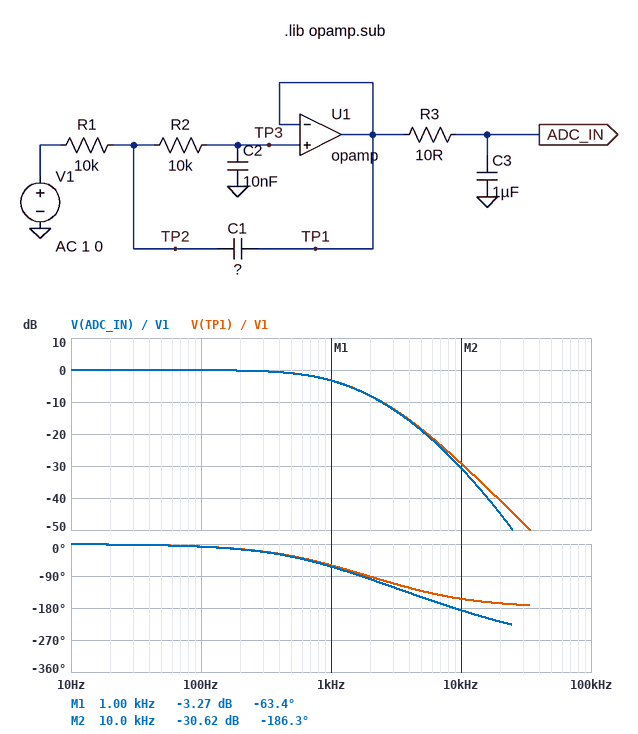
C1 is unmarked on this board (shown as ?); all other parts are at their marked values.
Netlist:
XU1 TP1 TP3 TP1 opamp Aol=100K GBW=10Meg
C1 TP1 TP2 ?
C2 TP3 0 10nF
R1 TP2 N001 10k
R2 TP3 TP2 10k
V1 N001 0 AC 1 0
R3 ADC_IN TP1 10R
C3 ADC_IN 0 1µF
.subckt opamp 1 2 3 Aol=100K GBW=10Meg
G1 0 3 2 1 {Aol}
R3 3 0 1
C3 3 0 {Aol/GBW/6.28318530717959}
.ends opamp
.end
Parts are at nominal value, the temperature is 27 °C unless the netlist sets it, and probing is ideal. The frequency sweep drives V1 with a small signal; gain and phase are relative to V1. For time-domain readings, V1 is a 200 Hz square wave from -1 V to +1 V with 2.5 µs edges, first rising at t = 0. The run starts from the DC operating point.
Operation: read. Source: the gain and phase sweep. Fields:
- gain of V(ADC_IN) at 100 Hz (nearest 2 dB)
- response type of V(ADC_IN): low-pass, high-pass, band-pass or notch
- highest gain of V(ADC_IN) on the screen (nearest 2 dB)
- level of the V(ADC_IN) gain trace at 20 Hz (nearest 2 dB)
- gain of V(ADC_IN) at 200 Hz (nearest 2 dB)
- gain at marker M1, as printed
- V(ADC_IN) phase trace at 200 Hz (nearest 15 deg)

0 dB
low-pass
0 dB
0 dB
0 dB
-3.27 dB
-15 deg
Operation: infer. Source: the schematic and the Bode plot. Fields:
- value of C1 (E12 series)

6.8 nF
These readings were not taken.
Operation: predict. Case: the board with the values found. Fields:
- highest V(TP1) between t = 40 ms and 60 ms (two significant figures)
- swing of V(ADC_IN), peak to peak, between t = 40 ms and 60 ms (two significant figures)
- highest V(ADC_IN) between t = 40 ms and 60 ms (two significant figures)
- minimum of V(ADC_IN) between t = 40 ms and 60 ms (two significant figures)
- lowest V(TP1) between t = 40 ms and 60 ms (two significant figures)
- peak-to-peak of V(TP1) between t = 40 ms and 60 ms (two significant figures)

1.0 V
2.0 V
1.0 V
-1.0 V
-1.0 V
2.0 V
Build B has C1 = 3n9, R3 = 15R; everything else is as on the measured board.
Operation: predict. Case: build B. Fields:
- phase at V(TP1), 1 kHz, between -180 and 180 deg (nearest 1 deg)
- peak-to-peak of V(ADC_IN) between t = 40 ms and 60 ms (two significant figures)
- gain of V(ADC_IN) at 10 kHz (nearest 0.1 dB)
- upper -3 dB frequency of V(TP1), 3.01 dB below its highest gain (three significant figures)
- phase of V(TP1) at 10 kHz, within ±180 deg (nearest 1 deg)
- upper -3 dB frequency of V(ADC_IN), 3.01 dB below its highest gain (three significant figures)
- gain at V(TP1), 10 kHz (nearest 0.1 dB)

-56 deg
2.0 V
-28.4 dB
881 Hz
-139 deg
875 Hz
-25.6 dB
